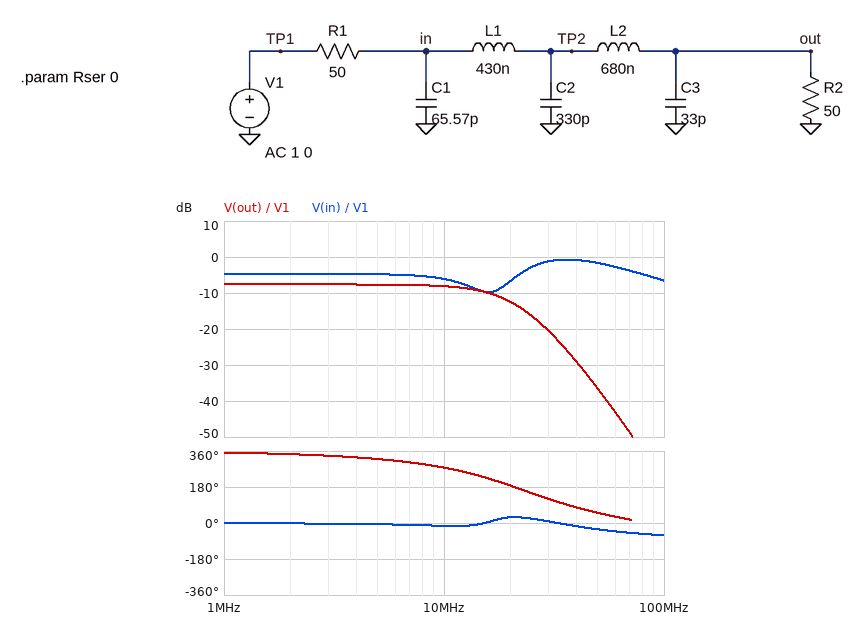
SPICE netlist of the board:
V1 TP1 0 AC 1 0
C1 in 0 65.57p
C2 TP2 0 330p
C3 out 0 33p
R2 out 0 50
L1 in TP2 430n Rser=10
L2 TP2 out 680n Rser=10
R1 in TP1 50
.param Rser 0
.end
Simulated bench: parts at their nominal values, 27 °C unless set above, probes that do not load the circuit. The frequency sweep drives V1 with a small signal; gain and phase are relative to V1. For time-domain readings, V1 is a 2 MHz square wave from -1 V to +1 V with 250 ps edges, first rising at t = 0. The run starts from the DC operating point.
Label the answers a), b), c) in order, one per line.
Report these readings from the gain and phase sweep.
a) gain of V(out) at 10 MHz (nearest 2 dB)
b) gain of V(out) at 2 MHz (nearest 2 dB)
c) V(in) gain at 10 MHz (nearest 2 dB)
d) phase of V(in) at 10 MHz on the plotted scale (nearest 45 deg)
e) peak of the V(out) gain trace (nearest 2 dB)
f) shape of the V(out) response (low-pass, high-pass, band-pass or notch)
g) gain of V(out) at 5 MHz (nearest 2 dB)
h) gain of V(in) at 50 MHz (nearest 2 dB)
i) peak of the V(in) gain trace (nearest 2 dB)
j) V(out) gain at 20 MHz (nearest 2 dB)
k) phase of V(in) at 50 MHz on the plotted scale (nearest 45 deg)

a) -8 dB
b) -8 dB
c) -6 dB
d) 0 deg
e) -8 dB
f) low-pass
g) -8 dB
h) -2 dB
i) 0 dB
j) -12 dB
k) -45 deg
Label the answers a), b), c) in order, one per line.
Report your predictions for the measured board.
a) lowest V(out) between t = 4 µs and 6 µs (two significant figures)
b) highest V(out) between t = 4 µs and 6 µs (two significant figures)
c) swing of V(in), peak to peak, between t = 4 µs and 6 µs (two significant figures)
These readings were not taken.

a) -460 mV
b) 460 mV
c) 1.6 V
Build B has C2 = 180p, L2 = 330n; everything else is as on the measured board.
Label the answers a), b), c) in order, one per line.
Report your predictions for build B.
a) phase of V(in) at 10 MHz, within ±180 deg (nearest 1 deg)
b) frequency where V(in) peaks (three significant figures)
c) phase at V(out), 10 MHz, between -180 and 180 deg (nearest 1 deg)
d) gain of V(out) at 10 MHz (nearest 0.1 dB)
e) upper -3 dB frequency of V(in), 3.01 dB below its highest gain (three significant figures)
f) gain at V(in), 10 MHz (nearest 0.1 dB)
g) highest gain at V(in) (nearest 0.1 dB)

a) -5 deg
b) 41.2 MHz
c) -53 deg
d) -7.7 dB
e) 73.4 MHz
f) -5.1 dB
g) -1.1 dB
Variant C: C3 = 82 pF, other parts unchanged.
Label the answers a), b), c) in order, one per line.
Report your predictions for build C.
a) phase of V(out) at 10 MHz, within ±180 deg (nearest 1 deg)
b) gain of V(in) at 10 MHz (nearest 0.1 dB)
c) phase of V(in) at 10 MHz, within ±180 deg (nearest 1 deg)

a) -87 deg
b) -6.3 dB
c) -12 deg
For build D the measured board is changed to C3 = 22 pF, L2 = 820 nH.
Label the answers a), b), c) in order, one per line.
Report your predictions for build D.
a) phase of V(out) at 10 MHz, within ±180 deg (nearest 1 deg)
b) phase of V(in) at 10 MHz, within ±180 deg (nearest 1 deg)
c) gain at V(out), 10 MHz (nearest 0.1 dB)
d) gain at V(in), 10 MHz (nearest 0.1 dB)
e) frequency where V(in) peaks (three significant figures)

a) -88 deg
b) -17 deg
c) -8.2 dB
d) -5.8 dB
e) 36.0 MHz
